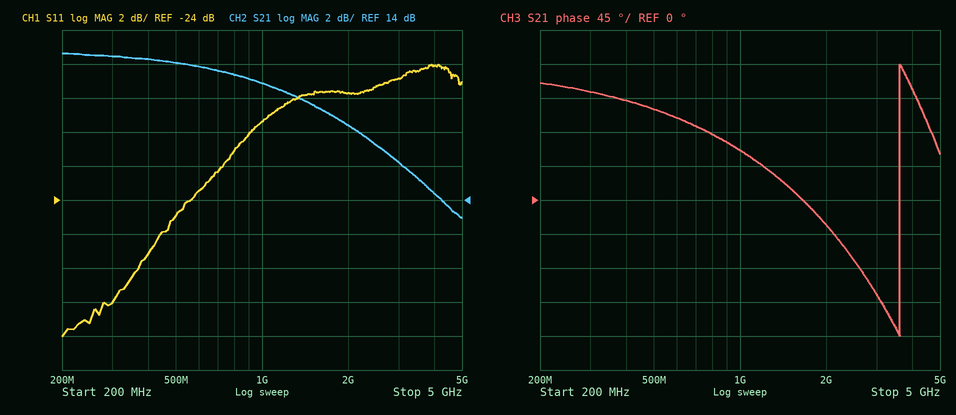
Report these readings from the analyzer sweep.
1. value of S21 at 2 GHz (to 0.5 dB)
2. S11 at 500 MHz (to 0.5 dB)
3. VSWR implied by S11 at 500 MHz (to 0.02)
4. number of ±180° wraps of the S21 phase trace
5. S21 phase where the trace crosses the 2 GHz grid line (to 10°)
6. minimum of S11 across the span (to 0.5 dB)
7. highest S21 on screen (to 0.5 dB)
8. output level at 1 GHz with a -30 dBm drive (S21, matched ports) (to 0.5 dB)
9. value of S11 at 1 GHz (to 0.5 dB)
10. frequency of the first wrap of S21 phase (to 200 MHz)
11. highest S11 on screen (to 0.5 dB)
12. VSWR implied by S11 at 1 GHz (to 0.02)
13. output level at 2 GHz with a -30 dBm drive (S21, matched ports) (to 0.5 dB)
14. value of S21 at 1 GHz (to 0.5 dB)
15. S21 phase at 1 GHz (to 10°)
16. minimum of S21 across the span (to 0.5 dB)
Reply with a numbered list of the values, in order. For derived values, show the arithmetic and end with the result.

1. 18.5 dB
2. -25.0 dB
3. |Γ| = 10^(-25/20) = 0.0562; VSWR = (1 + 0.0562)/(1 − 0.0562) ≈ 1.12
4. 1
5. -30°
6. -32.0 dB
7. 22.5 dB
8. -30 dBm + (21.0 dB) = -9.0 dBm
9. -19.5 dB
10. 3.6 GHz
11. -16.0 dB
12. |Γ| = 10^(-19.5/20) = 0.1059; VSWR = (1 + 0.1059)/(1 − 0.1059) ≈ 1.24
13. -30 dBm + (18.5 dB) = -11.5 dBm
14. 21.0 dB
15. 70°
16. 13.0 dB
